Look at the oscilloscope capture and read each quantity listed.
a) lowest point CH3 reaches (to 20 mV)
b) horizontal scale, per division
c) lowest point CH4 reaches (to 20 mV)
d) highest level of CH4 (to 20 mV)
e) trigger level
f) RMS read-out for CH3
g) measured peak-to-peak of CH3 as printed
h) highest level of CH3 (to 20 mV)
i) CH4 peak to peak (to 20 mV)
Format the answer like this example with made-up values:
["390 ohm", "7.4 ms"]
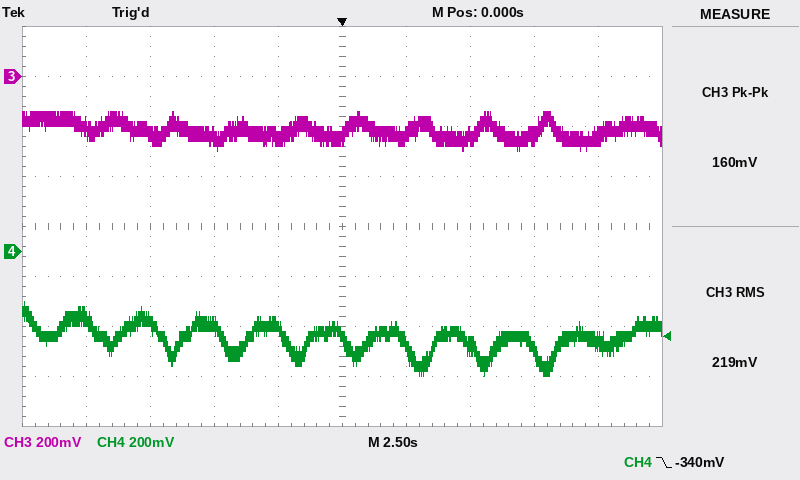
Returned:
["-300 mV", "2.5 s", "-500 mV", "-200 mV", "-340 mV", "219 mV", "160 mV", "-140 mV", "300 mV"]
